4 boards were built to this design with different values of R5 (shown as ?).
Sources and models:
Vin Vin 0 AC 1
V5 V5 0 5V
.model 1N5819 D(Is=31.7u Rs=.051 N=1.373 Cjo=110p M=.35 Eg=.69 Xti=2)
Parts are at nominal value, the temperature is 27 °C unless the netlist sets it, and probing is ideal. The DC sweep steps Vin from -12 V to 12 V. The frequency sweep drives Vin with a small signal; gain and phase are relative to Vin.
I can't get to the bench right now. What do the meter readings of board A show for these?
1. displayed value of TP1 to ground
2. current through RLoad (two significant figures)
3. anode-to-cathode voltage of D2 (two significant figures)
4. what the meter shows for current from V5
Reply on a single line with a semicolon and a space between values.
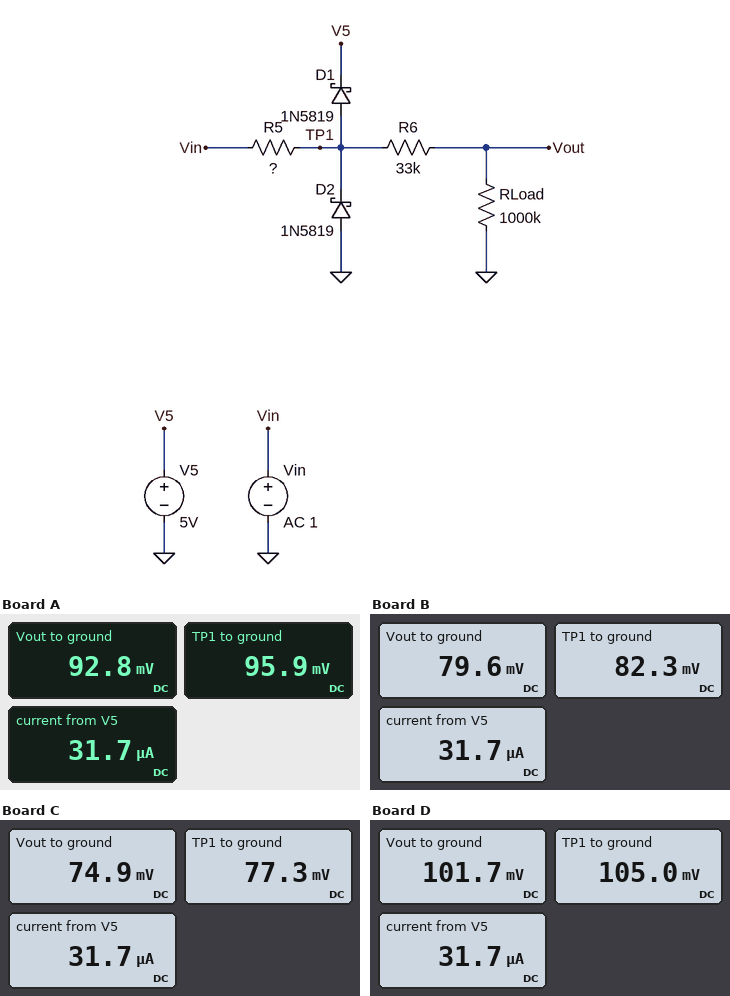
95.9 mV; 93 nA; -96 mV; 31.7 µA
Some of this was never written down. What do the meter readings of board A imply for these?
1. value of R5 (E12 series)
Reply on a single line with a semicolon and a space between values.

47 kΩ
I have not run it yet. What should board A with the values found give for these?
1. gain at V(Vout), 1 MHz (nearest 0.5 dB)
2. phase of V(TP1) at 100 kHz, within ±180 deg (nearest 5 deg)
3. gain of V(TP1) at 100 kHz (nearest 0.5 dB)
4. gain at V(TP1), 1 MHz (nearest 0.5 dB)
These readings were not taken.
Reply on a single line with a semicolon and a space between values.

-34.0 dB; -50 deg; -16.0 dB; -34.0 dB
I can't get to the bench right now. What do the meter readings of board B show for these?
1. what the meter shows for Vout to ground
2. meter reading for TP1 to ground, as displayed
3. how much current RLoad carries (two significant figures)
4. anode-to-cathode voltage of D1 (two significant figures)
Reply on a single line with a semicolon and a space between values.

79.6 mV; 82.3 mV; 80 nA; -4.9 V
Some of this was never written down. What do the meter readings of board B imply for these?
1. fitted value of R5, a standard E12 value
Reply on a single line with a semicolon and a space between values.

27 kΩ
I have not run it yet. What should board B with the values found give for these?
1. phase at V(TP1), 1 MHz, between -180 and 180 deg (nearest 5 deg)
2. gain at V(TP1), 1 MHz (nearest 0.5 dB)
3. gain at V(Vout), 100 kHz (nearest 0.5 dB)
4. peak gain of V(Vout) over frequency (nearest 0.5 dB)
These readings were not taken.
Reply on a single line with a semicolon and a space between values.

-85 deg; -29.0 dB; -13.0 dB; -11.0 dB
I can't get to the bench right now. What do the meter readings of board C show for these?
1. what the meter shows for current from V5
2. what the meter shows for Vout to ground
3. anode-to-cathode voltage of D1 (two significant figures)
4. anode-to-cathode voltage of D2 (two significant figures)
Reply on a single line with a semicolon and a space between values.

31.7 µA; 74.9 mV; -4.9 V; -77 mV
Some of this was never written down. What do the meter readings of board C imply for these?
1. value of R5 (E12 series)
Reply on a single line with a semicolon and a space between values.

22 kΩ
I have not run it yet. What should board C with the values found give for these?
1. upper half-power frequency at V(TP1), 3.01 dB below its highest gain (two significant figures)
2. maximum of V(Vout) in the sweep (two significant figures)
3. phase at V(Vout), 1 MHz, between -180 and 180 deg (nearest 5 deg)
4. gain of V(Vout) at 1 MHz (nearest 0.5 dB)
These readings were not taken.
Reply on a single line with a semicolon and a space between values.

140 kHz; 4.9 V; -80 deg; -27.5 dB
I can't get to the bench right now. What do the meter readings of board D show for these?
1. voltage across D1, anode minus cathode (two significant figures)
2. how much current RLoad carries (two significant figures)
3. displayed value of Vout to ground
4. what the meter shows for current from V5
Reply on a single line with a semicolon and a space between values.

-4.9 V; 100 nA; 101.7 mV; 31.7 µA
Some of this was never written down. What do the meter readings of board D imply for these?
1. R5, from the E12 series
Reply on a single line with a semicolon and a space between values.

68 kΩ
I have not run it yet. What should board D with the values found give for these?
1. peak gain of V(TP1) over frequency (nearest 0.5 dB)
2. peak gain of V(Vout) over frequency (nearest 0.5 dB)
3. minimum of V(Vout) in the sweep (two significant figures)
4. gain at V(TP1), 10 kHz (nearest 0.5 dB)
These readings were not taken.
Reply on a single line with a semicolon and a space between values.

-12.5 dB; -13.0 dB; -59 mV; -12.5 dB
